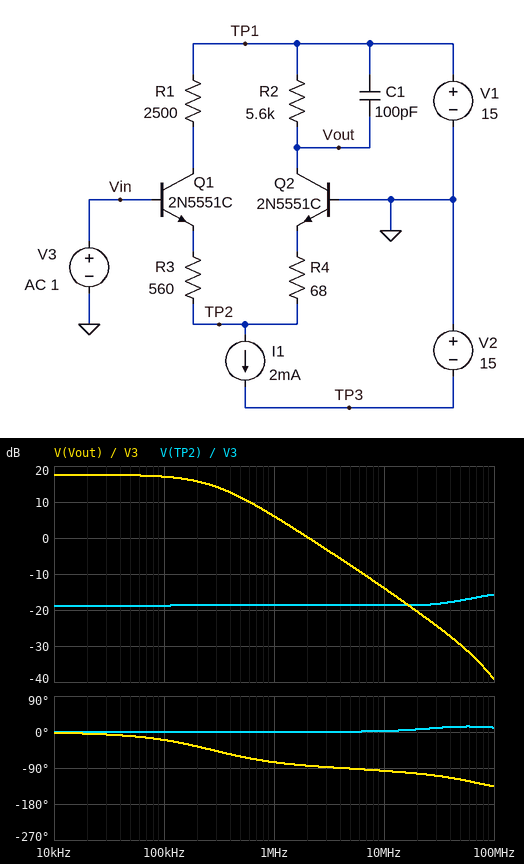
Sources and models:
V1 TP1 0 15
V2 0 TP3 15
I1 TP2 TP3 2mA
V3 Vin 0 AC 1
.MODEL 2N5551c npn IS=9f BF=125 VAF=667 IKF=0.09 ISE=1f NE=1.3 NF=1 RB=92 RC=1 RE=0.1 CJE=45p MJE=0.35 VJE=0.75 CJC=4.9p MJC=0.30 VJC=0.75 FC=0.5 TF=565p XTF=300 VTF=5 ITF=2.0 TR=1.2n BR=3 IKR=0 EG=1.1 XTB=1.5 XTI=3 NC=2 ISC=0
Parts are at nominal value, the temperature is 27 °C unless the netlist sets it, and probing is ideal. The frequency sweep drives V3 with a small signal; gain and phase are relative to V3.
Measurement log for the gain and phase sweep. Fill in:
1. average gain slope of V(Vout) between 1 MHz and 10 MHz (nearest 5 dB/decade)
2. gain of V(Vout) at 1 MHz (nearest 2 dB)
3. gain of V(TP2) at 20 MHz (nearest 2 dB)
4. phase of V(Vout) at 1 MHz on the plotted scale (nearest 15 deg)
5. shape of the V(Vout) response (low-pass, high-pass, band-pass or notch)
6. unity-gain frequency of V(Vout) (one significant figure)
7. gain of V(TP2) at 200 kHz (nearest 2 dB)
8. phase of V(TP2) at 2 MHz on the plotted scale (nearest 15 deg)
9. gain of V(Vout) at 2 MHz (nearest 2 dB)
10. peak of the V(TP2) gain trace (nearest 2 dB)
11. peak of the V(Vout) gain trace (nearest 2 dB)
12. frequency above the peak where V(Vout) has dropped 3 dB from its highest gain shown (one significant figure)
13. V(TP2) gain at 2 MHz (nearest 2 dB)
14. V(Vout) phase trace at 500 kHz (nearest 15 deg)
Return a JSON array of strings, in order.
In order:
["-20 dB/decade", "6 dB", "-18 dB", "-75 deg", "low-pass", "2 MHz", "-18 dB", "0 deg", "0 dB", "-16 dB", "18 dB", "300 kHz", "-18 dB", "-60 deg"]
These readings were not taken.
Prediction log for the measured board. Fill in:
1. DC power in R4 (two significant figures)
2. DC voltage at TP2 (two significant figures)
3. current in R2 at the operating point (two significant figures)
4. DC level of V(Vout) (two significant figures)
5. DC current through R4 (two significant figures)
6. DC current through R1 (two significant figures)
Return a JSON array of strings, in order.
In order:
["200 µW", "-790 mV", "1.7 mA", "5.5 V", "1.7 mA", "290 µA"]
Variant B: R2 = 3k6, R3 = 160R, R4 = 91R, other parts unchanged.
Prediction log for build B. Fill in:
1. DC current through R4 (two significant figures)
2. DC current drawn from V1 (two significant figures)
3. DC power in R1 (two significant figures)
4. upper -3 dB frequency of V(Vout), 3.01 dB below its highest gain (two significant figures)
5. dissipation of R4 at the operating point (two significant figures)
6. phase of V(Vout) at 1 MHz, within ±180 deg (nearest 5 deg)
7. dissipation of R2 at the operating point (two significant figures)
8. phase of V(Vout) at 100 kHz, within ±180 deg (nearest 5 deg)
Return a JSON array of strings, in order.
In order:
["1.2 mA", "2.0 mA", "1.5 mW", "430 kHz", "140 µW", "-70 deg", "5.3 mW", "-15 deg"]
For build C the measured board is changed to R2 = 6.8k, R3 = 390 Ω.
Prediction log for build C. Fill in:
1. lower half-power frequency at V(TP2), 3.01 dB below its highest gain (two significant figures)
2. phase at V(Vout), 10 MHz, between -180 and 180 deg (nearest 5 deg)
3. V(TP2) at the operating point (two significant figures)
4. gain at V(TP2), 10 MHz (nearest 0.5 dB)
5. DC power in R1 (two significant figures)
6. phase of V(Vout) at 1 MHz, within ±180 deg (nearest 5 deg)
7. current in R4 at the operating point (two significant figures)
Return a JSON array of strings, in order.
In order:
["36 MHz", "-100 deg", "-780 mV", "-16.0 dB", "360 µW", "-80 deg", "1.6 mA"]
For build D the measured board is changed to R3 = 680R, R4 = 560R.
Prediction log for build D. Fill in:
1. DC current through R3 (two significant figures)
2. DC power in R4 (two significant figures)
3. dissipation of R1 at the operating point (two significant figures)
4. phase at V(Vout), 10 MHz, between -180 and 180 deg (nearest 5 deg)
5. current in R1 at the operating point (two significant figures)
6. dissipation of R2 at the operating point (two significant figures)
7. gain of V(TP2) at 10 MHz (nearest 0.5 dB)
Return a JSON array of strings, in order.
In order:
["910 µA", "670 µW", "2.0 mW", "-100 deg", "900 µA", "6.6 mW", "-7.0 dB"]
